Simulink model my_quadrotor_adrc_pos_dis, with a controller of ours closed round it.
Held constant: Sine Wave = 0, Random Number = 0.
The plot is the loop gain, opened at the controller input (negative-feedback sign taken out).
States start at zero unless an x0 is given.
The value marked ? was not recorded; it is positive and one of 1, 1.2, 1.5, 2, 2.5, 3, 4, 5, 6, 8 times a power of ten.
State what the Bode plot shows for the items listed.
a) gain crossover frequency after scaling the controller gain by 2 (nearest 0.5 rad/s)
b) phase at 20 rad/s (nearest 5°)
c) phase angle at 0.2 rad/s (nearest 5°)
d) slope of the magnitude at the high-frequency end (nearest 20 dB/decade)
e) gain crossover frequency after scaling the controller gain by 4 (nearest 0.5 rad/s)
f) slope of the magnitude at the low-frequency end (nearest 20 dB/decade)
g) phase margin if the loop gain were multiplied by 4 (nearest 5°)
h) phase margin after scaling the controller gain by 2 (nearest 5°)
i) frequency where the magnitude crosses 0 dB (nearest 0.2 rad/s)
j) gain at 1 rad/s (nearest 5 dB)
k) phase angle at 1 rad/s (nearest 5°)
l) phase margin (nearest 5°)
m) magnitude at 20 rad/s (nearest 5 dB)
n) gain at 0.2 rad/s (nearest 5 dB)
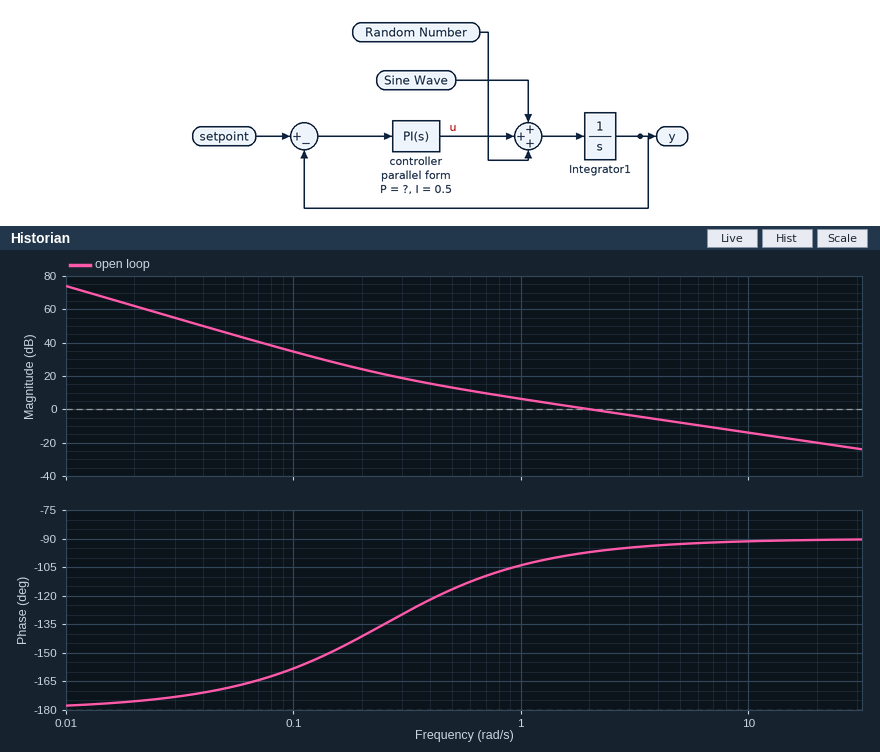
4.0 rad/s
-90°
-140°
-20 dB/decade
8.0 rad/s
-40 dB/decade
90°
85°
2.0 rad/s
5 dB
-105°
85°
-20 dB
25 dB
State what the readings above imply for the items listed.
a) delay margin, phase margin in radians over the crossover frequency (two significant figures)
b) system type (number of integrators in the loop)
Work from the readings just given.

0.74 s
2
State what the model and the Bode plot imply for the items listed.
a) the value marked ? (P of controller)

2
